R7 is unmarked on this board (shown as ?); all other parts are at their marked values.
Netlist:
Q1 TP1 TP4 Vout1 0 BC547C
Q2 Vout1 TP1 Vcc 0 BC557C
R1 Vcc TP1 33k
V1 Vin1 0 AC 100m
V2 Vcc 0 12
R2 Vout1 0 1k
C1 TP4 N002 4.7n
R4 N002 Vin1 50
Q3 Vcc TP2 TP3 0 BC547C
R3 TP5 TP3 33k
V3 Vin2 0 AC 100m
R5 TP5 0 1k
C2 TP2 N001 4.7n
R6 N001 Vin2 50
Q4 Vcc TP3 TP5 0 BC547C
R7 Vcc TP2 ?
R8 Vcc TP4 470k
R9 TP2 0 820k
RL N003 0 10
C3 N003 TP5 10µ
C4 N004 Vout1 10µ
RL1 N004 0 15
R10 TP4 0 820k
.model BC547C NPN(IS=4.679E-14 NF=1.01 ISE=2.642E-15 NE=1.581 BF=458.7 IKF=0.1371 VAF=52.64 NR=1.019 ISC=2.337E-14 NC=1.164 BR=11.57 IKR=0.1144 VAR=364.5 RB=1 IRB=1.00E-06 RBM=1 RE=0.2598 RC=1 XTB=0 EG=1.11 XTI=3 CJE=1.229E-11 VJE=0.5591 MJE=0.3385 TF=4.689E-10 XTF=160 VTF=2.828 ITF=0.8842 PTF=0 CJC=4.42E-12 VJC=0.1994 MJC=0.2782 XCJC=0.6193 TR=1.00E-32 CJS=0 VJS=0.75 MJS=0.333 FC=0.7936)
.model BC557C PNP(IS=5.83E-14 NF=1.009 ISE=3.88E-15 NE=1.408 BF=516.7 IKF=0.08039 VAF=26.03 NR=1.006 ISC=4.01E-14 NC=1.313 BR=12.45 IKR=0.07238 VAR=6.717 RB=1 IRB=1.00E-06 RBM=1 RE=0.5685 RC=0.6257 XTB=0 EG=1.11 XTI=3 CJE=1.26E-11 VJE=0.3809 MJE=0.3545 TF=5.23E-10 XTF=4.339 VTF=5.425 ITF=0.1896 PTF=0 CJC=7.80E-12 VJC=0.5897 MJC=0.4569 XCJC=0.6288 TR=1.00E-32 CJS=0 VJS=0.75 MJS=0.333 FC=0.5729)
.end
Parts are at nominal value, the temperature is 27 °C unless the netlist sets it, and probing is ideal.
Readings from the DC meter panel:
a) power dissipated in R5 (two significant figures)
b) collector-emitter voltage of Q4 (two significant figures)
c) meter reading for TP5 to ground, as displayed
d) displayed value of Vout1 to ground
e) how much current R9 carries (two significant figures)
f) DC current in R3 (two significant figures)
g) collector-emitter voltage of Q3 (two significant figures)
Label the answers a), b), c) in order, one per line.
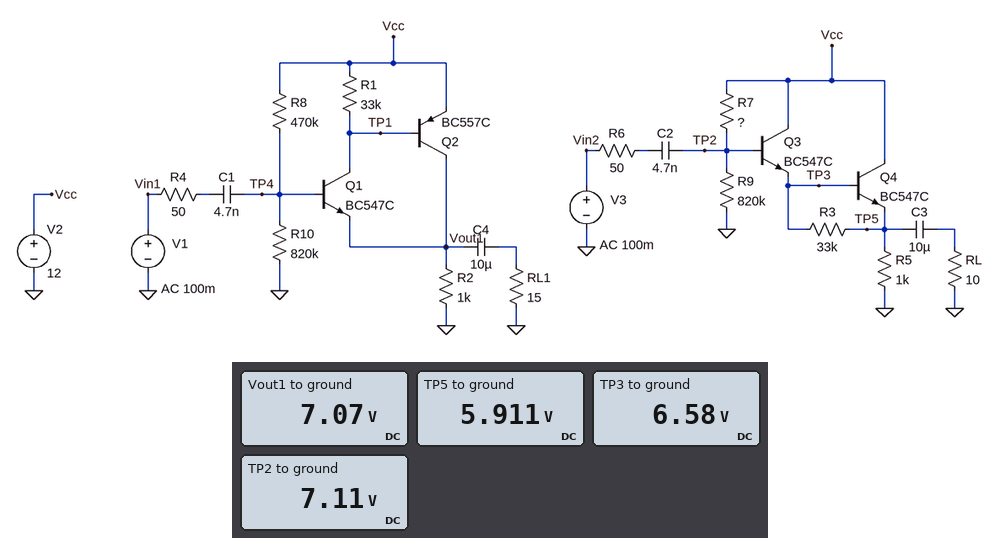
a) 35 mW
b) 6.1 V
c) 5.911 V
d) 7.07 V
e) 8.7 µA
f) 20 µA
g) 5.4 V
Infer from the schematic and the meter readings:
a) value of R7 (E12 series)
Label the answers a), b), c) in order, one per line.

a) 560 kΩ
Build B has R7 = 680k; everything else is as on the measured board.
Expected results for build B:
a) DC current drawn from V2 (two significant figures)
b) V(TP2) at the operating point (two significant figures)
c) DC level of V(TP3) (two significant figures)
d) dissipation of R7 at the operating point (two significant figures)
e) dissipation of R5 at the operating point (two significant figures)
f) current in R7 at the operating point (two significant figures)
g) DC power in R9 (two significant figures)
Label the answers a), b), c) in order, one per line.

a) 12 mA
b) 6.5 V
c) 6.0 V
d) 44 µW
e) 29 mW
f) 8.0 µA
g) 52 µW
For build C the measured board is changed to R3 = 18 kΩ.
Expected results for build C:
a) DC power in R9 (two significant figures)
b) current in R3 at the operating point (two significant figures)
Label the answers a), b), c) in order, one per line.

a) 61 µW
b) 37 µA
